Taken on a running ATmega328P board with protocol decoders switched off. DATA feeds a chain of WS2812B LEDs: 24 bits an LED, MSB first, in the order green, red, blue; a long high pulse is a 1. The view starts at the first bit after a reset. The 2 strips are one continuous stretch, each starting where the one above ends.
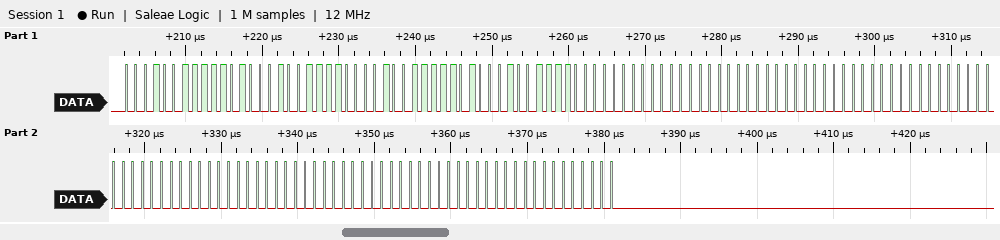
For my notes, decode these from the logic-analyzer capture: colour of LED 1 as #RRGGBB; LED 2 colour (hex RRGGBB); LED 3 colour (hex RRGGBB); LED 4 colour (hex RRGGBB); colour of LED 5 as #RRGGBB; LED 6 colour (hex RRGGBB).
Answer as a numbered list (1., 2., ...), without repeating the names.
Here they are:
1. #E8139E
2. #E8139E
3. #000000
4. #000000
5. #000000
6. #000000
